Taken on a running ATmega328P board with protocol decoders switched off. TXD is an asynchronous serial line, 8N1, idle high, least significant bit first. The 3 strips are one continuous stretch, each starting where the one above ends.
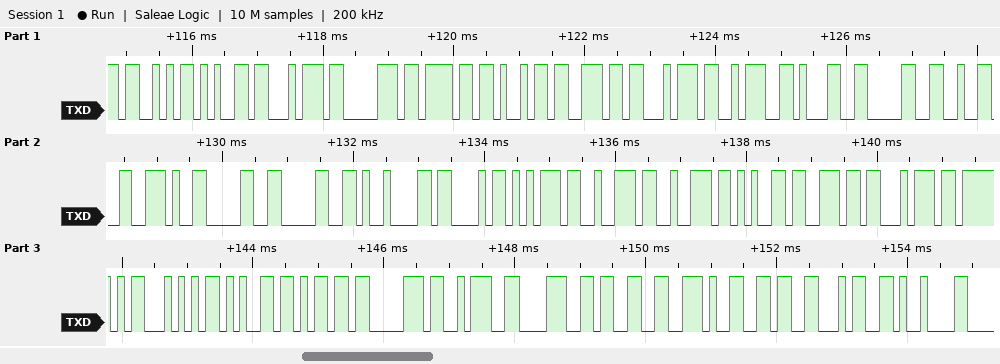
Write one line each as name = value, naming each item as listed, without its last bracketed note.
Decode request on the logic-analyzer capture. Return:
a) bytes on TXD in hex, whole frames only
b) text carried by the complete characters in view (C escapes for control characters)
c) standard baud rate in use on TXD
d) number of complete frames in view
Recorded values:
bytes on TXD in hex, whole frames only = 53 65 74 70 6F 69 6E 74 3A 31 30 32 2E 30 30 09 43 75 72 72 65 6E 74 5F 54 65 6D 70 3A 38 33 2E 36 34 09
text carried by the complete characters in view = "Setpoint:102.00\tCurrent_Temp:83.64\t"
standard baud rate in use on TXD = 9600 baud
number of complete frames in view = 35
